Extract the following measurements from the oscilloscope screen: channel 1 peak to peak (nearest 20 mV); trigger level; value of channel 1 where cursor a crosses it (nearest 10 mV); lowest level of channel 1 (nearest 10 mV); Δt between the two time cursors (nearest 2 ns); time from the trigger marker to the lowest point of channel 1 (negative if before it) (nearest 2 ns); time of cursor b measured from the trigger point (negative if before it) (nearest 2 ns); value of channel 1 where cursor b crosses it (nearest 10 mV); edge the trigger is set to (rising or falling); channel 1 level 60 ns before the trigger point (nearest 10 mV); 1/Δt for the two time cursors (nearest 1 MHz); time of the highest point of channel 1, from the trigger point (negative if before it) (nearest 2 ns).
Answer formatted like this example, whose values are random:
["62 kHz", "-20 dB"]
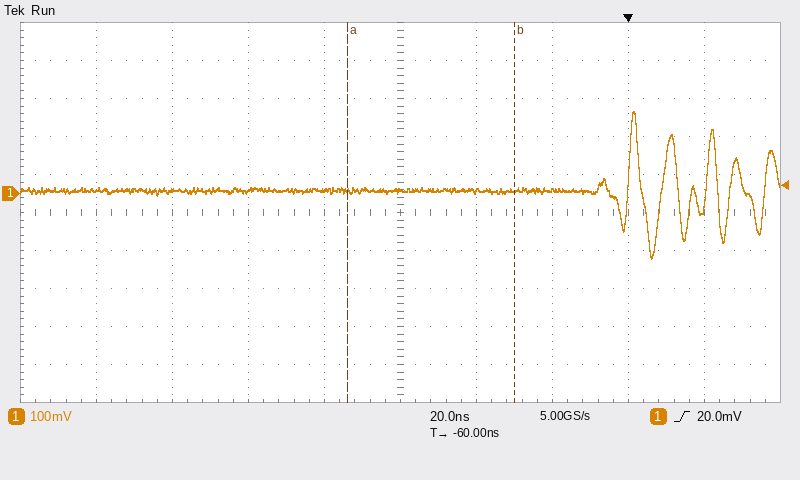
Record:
["380 mV", "20.0 mV", "10 mV", "-170 mV", "44 ns", "+6 ns", "-30 ns", "10 mV", "rising", "10 mV", "23 MHz", "+2 ns"]
